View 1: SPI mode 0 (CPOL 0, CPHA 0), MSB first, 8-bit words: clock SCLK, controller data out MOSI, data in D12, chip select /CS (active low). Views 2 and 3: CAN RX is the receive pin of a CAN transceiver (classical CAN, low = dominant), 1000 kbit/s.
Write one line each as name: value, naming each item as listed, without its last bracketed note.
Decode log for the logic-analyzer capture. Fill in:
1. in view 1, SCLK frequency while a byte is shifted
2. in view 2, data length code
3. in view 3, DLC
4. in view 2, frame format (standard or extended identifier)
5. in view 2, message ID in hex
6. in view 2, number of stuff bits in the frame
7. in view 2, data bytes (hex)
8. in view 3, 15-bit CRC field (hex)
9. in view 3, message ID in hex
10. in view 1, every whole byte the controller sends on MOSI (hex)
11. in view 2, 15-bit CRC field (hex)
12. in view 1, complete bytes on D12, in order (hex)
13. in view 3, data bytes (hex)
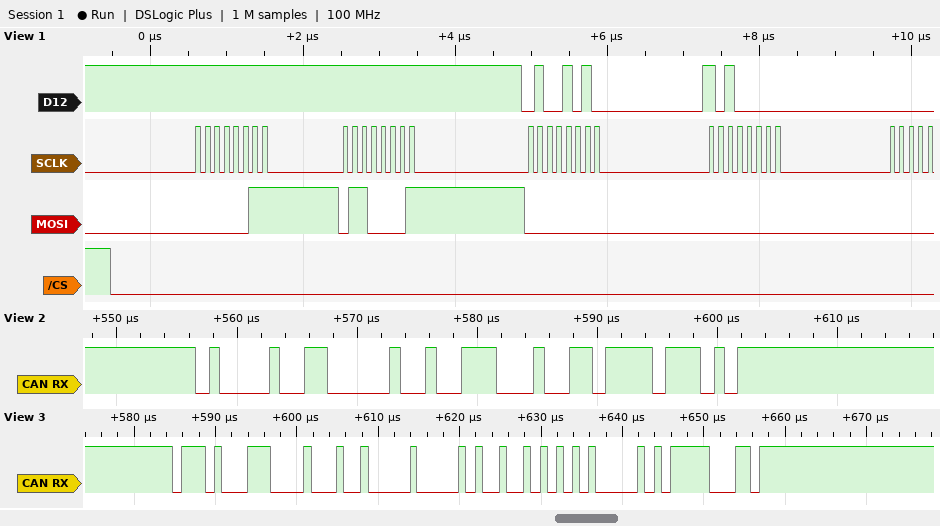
in view 1, SCLK frequency while a byte is shifted: 8 MHz
in view 2, data length code: 1
in view 3, DLC: 4
in view 2, frame format: standard
in view 2, message ID in hex: 0x426
in view 2, number of stuff bits in the frame: 1
in view 2, data bytes: 38
in view 3, 15-bit CRC field: 0x02F9
in view 3, message ID in hex: 0x747
in view 1, every whole byte the controller sends on MOSI: 03 61 00 00
in view 2, 15-bit CRC field: 0x4DEE
in view 1, complete bytes on D12, in order: FF FF 4A A0
in view 3, data bytes: 48 00 92 AA
